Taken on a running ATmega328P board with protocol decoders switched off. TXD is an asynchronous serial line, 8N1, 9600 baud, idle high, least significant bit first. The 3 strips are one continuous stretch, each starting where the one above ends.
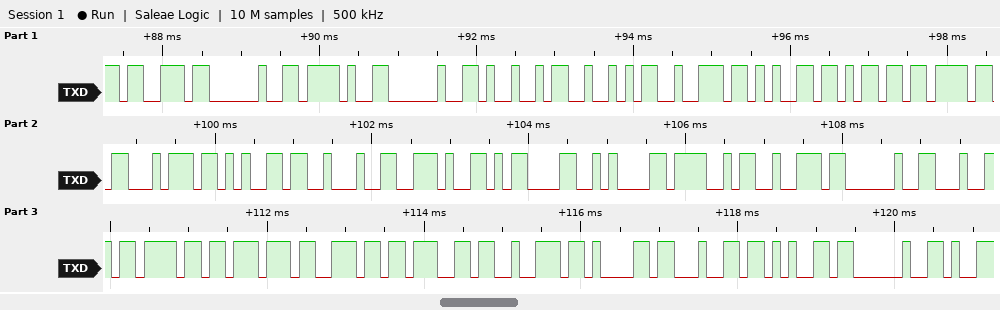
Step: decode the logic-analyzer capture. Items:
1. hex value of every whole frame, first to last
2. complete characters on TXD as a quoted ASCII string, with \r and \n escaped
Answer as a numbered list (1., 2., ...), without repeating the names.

1. 0x73 0x20 0x2F 0x20 0x49 0x52 0x72 0x65 0x6D 0x6F 0x74 0x65 0x22 0x2E 0x0D 0x0A 0x4F 0x72 0x20 0x64 0x6F 0x77 0x6E 0x67 0x72 0x61 0x64 0x65 0x20
2. "s / IRremote\".\r\nOr downgrade "
